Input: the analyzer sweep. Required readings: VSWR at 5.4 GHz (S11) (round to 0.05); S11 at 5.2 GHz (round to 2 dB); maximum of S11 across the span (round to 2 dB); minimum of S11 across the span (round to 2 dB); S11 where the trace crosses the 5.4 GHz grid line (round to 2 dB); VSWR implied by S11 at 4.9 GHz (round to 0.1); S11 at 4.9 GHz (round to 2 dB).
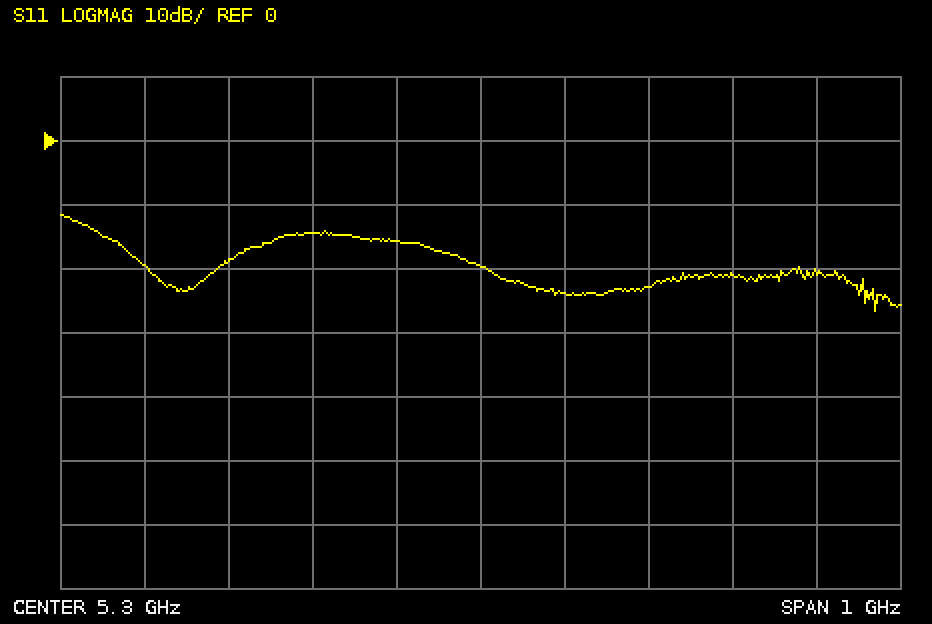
1.15
-16 dB
-12 dB
-26 dB
-24 dB
1.2
-20 dB
